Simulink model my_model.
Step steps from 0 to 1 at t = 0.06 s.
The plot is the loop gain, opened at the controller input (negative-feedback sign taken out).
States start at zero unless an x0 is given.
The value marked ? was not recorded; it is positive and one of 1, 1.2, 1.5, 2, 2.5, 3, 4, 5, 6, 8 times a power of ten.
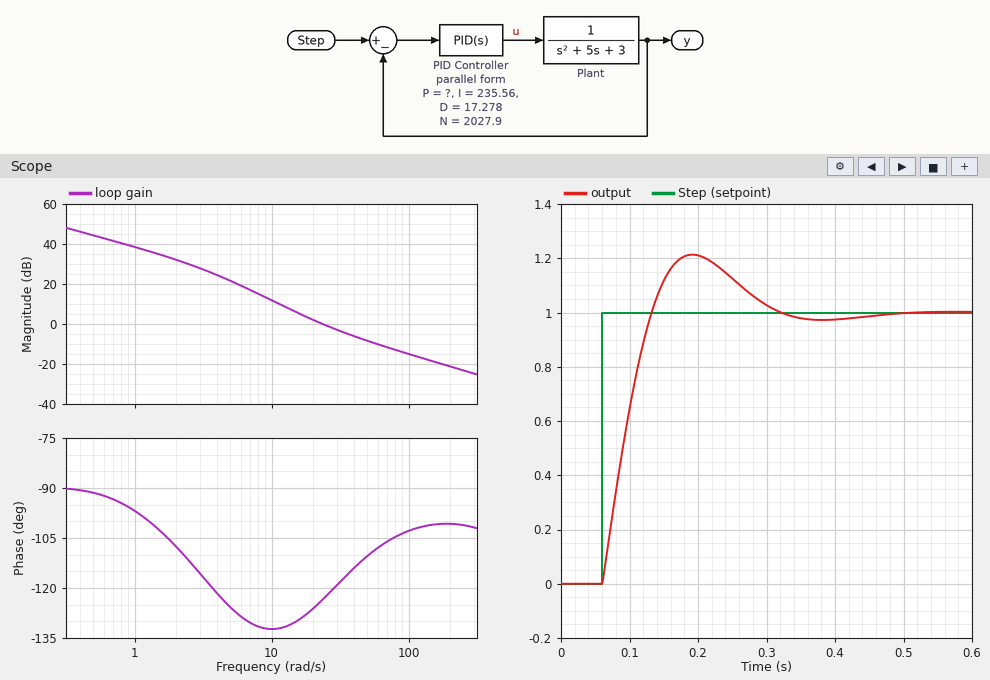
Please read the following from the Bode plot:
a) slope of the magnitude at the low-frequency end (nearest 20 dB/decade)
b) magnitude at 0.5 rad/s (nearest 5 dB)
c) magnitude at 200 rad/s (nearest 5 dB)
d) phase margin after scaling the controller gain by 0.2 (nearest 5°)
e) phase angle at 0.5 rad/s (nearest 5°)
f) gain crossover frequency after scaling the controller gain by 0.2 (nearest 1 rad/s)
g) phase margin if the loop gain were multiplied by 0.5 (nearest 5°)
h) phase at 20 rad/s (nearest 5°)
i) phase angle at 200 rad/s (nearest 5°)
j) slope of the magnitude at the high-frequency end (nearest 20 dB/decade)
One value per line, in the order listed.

-20 dB/decade
45 dB
-20 dB
50°
-90°
9 rad/s
50°
-125°
-100°
-20 dB/decade
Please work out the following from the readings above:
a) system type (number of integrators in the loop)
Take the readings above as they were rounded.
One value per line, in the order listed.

1
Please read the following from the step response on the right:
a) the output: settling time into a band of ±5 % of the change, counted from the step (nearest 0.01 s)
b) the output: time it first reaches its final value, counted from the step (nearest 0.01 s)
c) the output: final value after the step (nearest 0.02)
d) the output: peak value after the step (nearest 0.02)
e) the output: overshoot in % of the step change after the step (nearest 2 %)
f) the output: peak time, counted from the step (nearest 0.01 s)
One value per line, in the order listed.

0.23 s
0.07 s
1.00
1.22
22 %
0.13 s
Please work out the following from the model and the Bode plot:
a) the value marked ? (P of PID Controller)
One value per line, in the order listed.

400
